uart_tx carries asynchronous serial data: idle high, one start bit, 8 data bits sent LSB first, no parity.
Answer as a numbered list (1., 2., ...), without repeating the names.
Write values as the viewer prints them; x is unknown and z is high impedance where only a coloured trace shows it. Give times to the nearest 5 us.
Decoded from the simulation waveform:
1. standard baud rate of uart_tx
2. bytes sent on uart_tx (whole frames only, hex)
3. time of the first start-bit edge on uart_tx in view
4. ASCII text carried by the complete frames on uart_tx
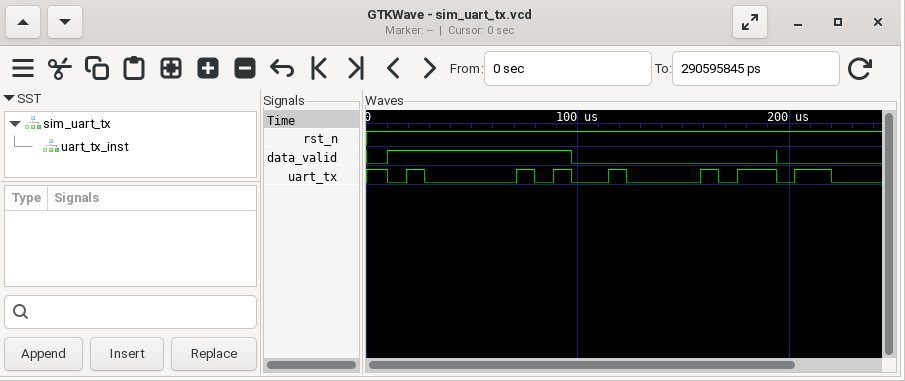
1. 115200 baud
2. 41, 42
3. 10 us
4. "AB"
